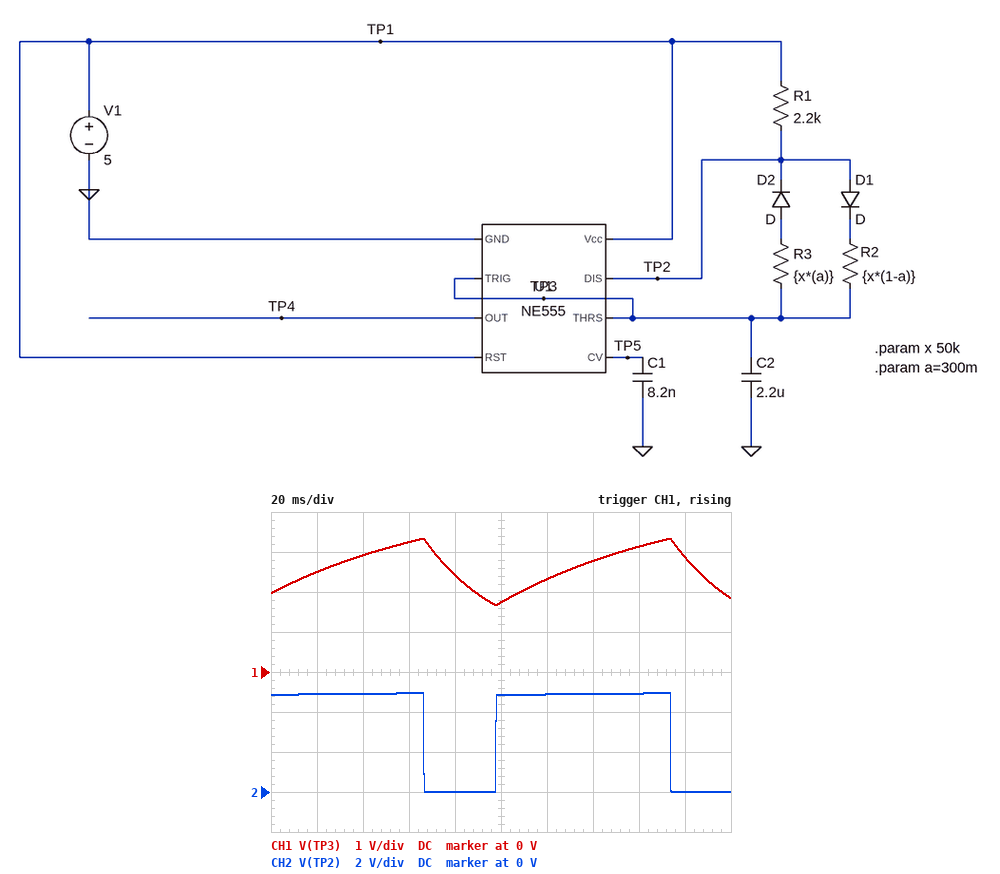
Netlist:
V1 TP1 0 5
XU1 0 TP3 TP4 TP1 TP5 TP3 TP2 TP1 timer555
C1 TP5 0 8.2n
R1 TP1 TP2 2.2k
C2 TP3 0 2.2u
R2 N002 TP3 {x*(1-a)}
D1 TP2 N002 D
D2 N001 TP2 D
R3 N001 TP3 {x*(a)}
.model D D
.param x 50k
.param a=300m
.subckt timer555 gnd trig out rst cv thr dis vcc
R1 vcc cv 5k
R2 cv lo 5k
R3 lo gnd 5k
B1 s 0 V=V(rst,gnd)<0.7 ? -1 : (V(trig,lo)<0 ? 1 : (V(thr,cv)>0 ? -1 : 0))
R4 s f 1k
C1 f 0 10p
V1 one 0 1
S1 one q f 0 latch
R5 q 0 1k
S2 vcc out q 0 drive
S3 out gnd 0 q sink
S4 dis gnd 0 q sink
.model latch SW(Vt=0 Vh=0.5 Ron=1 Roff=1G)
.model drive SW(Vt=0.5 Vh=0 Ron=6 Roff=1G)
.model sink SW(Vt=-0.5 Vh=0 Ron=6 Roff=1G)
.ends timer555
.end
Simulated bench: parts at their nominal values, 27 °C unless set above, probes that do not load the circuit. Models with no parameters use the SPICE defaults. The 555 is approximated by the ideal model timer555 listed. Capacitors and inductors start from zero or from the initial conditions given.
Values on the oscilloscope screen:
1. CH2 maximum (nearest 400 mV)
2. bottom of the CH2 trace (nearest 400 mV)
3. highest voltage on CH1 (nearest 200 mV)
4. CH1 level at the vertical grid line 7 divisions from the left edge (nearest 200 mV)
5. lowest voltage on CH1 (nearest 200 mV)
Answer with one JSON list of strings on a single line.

["4.8 V", "0 V", "3.4 V", "2.8 V", "1.6 V"]
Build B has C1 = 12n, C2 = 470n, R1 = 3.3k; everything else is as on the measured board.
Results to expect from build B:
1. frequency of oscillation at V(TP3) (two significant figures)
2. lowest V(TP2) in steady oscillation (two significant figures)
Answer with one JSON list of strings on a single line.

["43 Hz", "9.5 mV"]
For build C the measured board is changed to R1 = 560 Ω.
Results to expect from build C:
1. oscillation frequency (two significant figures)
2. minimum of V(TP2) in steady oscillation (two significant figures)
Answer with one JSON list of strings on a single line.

["9.6 Hz", "53 mV"]
